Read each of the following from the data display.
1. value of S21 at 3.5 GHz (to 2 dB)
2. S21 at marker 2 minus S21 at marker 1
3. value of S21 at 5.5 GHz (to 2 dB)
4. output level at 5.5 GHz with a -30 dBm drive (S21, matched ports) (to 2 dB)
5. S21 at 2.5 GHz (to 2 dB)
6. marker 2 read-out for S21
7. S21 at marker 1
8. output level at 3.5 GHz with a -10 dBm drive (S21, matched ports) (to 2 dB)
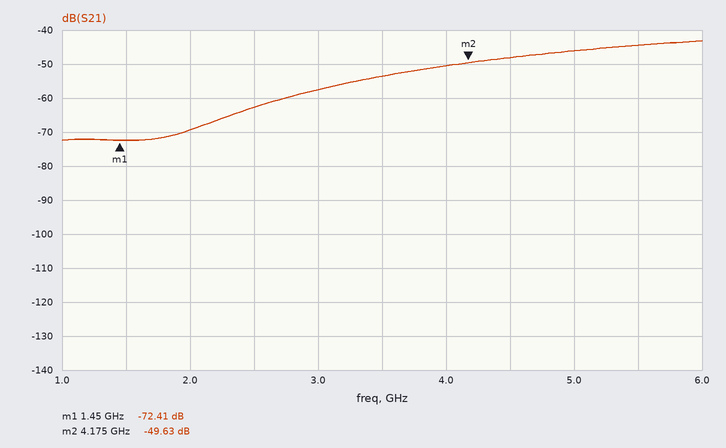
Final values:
-54 dB
22.78 dB
-44 dB
-74 dBm
-62 dB
-49.63 dB
-72.41 dB
-64 dBm
